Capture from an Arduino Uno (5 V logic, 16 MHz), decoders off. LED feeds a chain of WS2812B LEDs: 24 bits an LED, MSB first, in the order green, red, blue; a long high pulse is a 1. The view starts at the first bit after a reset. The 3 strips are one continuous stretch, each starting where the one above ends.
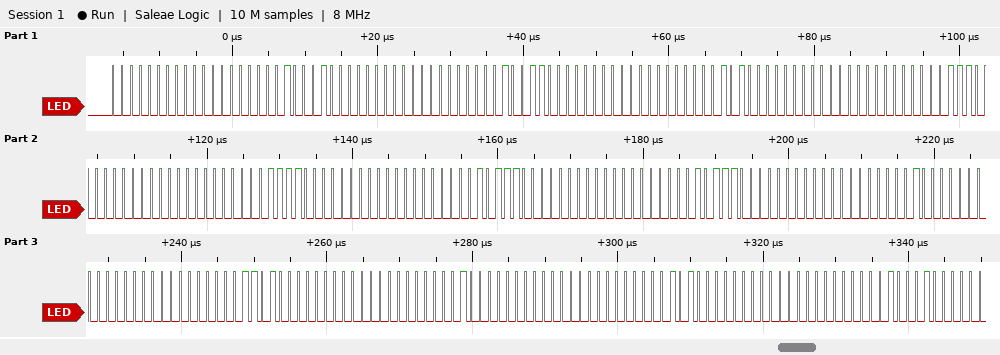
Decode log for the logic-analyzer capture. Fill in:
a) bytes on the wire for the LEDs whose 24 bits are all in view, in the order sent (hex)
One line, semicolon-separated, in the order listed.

00 00 11 00 00 13 00 00 14 00 00 0E 00 00 0F 00 00 17 00 00 17 00 00 10 00 00 0D 00 00 08 00 00 14 00 00 11
